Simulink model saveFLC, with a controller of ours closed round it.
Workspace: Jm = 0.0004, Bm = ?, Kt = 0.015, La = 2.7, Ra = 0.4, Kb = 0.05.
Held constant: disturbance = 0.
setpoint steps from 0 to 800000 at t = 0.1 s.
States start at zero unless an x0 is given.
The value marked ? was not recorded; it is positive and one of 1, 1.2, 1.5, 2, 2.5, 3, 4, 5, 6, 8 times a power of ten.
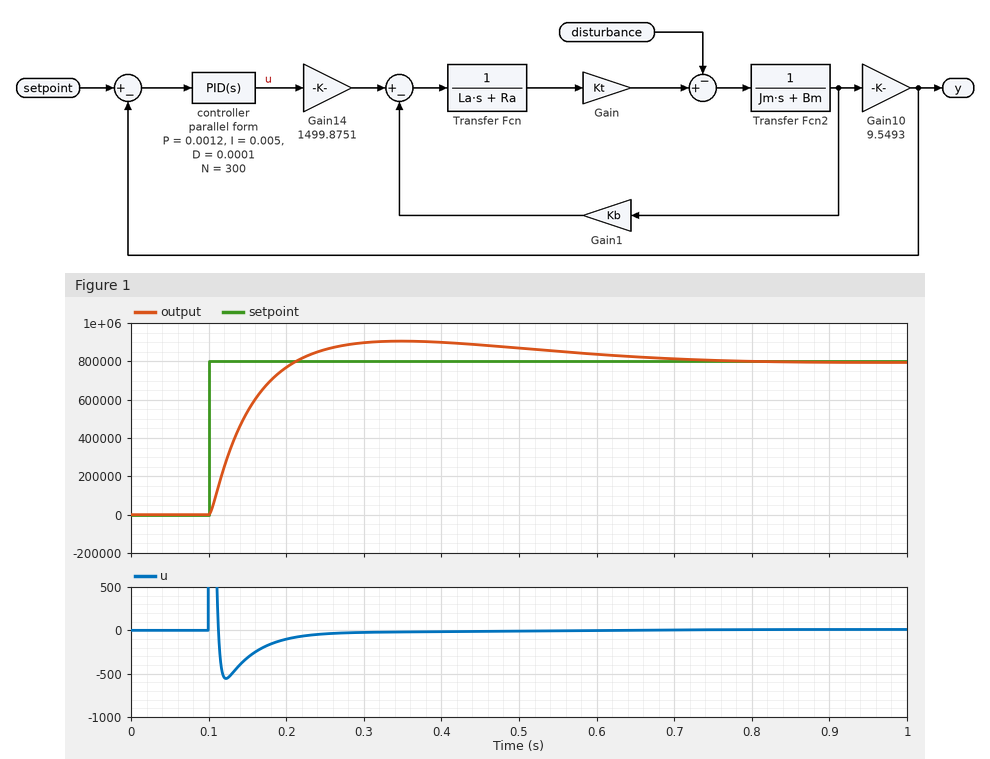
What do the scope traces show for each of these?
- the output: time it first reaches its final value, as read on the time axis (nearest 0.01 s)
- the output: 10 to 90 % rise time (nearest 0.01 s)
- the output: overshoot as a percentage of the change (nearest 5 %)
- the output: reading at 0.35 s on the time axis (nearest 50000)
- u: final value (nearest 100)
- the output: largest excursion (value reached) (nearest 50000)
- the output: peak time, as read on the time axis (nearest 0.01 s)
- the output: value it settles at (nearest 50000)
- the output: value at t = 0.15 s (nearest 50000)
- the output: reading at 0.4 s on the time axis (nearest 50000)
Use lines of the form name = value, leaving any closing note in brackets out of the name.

the output: time it first reaches its final value, as read on the time axis = 0.21 s
the output: 10 to 90 % rise time = 0.08 s
the output: overshoot as a percentage of the change = 15 %
the output: reading at 0.35 s on the time axis = 900000
u: final value = 0
the output: largest excursion (value reached) = 900000
the output: peak time, as read on the time axis = 0.35 s
the output: value it settles at = 800000
the output: value at t = 0.15 s = 550000
the output: reading at 0.4 s on the time axis = 900000
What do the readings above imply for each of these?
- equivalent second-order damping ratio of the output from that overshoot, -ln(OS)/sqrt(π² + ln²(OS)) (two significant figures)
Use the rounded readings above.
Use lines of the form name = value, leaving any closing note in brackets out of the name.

equivalent second-order damping ratio of the output from that overshoot, -ln(OS)/sqrt(π² + ln²(OS)) = 0.52
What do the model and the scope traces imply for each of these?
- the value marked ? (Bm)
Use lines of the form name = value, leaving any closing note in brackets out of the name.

the value marked ? = 0.004
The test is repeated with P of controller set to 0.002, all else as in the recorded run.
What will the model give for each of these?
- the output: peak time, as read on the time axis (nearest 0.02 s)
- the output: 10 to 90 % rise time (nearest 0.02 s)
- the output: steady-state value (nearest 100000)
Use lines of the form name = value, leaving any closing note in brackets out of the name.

the output: peak time, as read on the time axis = 0.24 s
the output: 10 to 90 % rise time = 0.06 s
the output: steady-state value = 800000
